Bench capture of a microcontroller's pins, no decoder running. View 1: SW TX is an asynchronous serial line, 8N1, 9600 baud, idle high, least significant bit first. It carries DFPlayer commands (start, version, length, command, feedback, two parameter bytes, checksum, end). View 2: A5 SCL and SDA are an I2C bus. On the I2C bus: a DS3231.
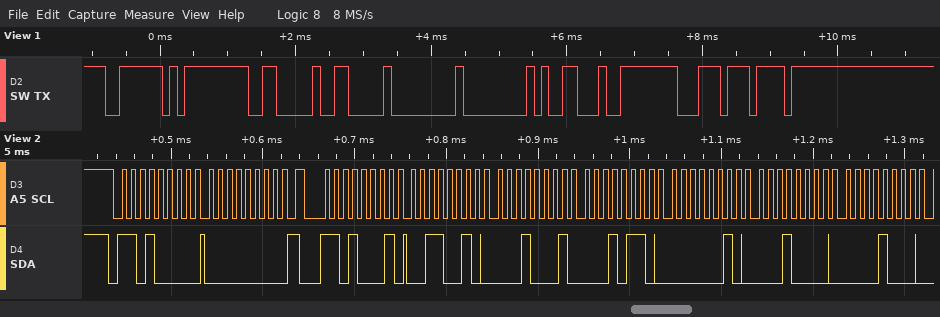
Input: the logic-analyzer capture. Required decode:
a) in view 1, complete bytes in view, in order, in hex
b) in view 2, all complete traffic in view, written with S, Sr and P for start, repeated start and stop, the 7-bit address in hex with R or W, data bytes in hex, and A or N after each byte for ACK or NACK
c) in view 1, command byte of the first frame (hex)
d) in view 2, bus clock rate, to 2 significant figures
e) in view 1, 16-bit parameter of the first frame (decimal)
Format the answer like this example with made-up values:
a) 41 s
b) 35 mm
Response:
a) 0x7E 0xFF 0x06 0x06 0x00 0x00 0x19 0xFE 0xDC 0xEF
b) S 68W A 00 A Sr 68R A 32 A 11 A 16 A 02 A 10 A 08 A
c) 0x06
d) 100 kHz
e) 25
